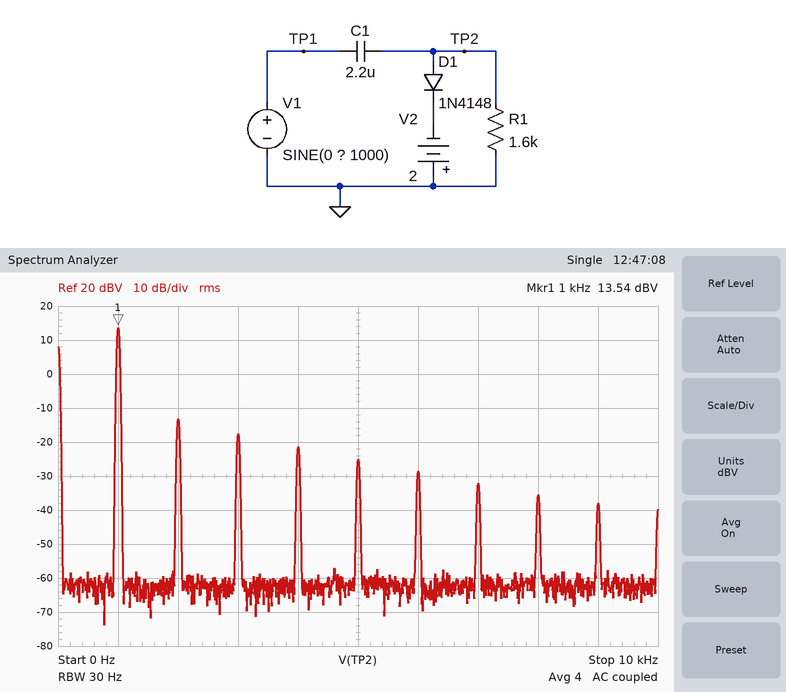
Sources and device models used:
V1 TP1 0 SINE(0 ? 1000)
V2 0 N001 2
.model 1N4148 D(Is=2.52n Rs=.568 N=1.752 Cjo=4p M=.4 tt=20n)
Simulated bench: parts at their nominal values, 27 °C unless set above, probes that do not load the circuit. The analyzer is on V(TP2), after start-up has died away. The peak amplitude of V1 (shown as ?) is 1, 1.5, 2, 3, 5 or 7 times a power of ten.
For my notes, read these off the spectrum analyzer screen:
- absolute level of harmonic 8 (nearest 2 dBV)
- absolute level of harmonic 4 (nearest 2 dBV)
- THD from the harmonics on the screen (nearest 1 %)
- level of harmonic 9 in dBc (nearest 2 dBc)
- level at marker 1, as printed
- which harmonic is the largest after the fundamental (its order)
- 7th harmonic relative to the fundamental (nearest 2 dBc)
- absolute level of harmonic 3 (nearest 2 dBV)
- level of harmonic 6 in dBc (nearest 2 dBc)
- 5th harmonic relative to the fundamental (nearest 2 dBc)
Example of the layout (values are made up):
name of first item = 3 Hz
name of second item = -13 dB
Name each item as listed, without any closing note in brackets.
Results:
absolute level of harmonic 8 = -36 dBV
absolute level of harmonic 4 = -22 dBV
THD from the harmonics on the screen = 6 %
level of harmonic 9 in dBc = -52 dBc
level at marker 1, as printed = 13.54 dBV
which harmonic is the largest after the fundamental = 2
7th harmonic relative to the fundamental = -46 dBc
absolute level of harmonic 3 = -18 dBV
level of harmonic 6 in dBc = -42 dBc
5th harmonic relative to the fundamental = -38 dBc
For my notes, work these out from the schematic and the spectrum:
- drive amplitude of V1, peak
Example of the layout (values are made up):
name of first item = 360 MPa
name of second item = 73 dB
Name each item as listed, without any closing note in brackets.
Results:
drive amplitude of V1, peak = 7 V
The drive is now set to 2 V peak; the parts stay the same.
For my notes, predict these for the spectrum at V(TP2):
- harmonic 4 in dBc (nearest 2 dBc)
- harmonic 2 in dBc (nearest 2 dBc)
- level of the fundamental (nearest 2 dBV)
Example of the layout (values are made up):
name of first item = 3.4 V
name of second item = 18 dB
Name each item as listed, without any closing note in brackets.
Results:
harmonic 4 in dBc = -34 dBc
harmonic 2 in dBc = -24 dBc
level of the fundamental = 2 dBV
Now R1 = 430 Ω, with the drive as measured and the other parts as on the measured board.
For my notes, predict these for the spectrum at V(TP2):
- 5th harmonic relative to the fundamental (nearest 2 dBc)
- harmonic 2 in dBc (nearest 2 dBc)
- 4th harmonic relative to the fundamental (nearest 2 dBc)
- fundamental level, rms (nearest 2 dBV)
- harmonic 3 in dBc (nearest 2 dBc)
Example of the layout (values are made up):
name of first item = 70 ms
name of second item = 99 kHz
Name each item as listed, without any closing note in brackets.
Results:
5th harmonic relative to the fundamental = -36 dBc
harmonic 2 in dBc = -18 dBc
4th harmonic relative to the fundamental = -30 dBc
fundamental level, rms = 12 dBV
harmonic 3 in dBc = -24 dBc
